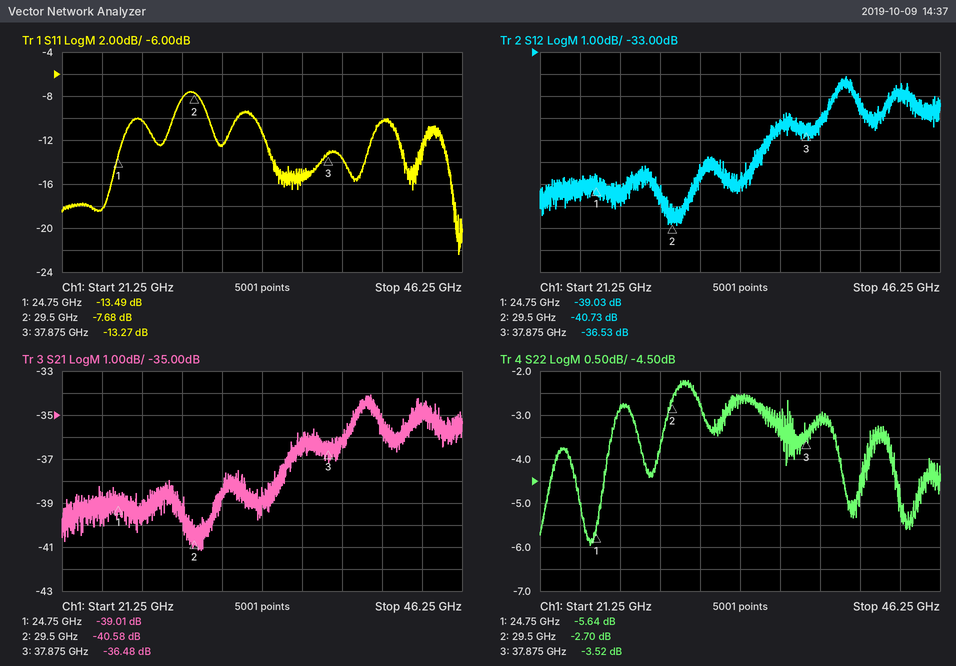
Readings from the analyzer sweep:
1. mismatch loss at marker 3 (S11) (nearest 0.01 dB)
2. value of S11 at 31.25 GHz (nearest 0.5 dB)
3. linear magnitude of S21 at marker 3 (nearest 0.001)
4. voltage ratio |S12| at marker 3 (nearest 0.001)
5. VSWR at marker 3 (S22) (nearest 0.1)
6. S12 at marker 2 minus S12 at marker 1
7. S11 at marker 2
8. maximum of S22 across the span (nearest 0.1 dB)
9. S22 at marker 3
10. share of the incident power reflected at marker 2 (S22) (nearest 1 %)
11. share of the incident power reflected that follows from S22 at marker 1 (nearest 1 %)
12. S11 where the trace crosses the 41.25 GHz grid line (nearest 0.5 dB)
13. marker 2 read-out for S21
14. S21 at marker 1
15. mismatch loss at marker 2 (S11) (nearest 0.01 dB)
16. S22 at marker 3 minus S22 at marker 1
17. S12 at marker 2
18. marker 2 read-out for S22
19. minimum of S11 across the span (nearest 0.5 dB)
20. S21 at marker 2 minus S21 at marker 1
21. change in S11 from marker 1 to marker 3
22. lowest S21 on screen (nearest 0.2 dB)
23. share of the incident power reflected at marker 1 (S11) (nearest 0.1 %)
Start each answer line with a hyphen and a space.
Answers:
- 0.21 dB
- -12.5 dB
- 0.015
- 0.015
- 5.0
- -1.70 dB
- -7.68 dB
- -2.2 dB
- -3.52 dB
- 54 %
- 27 %
- -10.5 dB
- -40.58 dB
- -39.01 dB
- 0.81 dB
- 2.12 dB
- -40.73 dB
- -2.70 dB
- -22.5 dB
- -1.57 dB
- 0.22 dB
- -41.2 dB
- 4.5 %
